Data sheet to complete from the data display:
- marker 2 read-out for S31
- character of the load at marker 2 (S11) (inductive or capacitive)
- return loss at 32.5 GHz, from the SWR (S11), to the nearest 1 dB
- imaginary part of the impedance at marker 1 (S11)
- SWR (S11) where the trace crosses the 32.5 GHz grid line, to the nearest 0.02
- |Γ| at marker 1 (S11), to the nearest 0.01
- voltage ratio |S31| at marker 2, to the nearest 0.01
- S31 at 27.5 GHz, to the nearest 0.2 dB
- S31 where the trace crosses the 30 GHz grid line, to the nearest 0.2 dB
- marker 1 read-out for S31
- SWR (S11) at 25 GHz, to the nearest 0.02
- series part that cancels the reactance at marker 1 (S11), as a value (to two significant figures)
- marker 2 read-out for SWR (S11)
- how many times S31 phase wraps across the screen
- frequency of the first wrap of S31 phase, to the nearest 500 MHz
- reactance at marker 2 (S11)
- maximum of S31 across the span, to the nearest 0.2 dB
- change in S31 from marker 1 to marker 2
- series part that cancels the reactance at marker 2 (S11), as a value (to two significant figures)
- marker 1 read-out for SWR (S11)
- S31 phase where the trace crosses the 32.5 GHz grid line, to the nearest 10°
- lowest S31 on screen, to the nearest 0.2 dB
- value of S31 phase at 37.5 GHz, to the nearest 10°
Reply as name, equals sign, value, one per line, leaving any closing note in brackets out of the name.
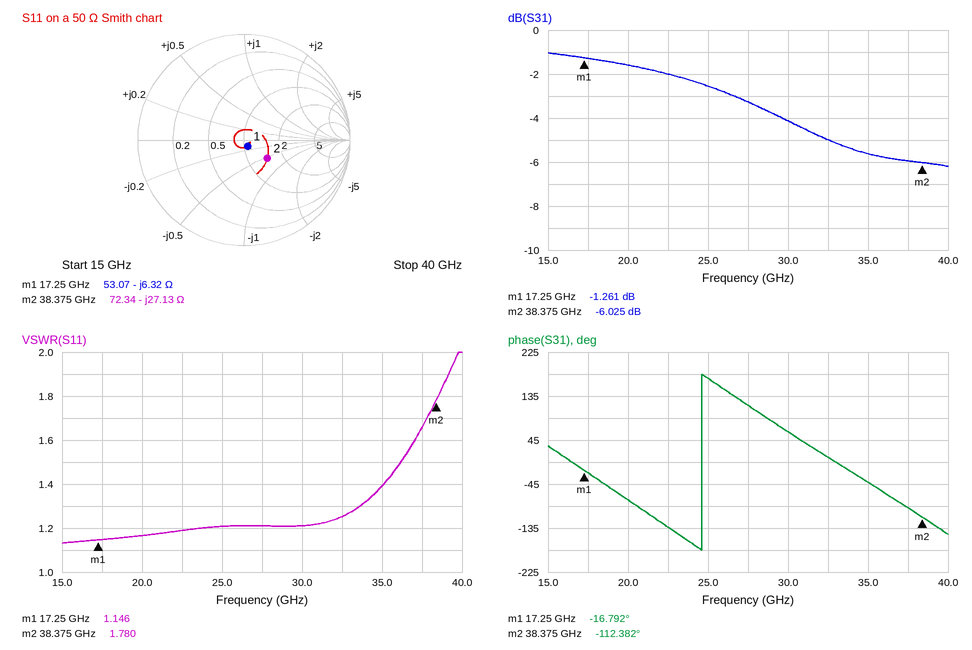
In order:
marker 2 read-out for S31 = -6.025 dB
character of the load at marker 2 (S11) = capacitive
return loss at 32.5 GHz, from the SWR (S11), to the nearest 1 dB = 19 dB
imaginary part of the impedance at marker 1 = -6.32 Ω
SWR (S11) where the trace crosses the 32.5 GHz grid line, to the nearest 0.02 = 1.26
|Γ| at marker 1 (S11), to the nearest 0.01 = 0.07
voltage ratio |S31| at marker 2, to the nearest 0.01 = 0.50
S31 at 27.5 GHz, to the nearest 0.2 dB = -3.2 dB
S31 where the trace crosses the 30 GHz grid line, to the nearest 0.2 dB = -4.2 dB
marker 1 read-out for S31 = -1.261 dB
SWR (S11) at 25 GHz, to the nearest 0.02 = 1.20
series part that cancels the reactance at marker 1 (S11), as a value = 58 pH
marker 2 read-out for SWR = 1.780
how many times S31 phase wraps across the screen = 1
frequency of the first wrap of S31 phase, to the nearest 500 MHz = 24.5 GHz
reactance at marker 2 = -27.13 Ω
maximum of S31 across the span, to the nearest 0.2 dB = -1.0 dB
change in S31 from marker 1 to marker 2 = -4.764 dB
series part that cancels the reactance at marker 2 (S11), as a value = 110 pH
marker 1 read-out for SWR = 1.146
S31 phase where the trace crosses the 32.5 GHz grid line, to the nearest 10° = 10°
lowest S31 on screen, to the nearest 0.2 dB = -6.2 dB
value of S31 phase at 37.5 GHz, to the nearest 10° = -90°
